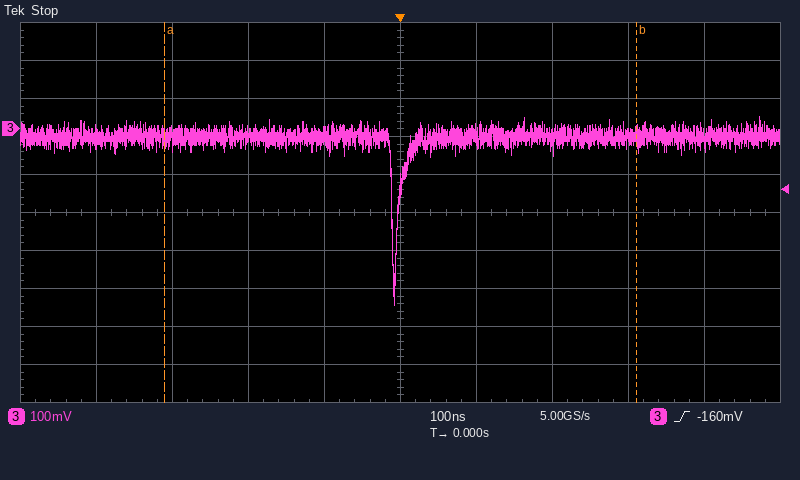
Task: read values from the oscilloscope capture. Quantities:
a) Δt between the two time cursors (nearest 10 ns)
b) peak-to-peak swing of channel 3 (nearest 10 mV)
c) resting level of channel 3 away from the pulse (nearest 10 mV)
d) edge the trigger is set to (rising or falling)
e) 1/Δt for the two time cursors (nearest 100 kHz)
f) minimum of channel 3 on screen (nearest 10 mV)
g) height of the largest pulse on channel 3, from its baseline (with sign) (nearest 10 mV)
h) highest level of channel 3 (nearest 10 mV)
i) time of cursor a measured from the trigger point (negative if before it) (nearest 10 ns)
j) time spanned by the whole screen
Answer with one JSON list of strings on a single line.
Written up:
["620 ns", "490 mV", "-20 mV", "rising", "1.6 MHz", "-460 mV", "-440 mV", "30 mV", "-310 ns", "1 µs"]
